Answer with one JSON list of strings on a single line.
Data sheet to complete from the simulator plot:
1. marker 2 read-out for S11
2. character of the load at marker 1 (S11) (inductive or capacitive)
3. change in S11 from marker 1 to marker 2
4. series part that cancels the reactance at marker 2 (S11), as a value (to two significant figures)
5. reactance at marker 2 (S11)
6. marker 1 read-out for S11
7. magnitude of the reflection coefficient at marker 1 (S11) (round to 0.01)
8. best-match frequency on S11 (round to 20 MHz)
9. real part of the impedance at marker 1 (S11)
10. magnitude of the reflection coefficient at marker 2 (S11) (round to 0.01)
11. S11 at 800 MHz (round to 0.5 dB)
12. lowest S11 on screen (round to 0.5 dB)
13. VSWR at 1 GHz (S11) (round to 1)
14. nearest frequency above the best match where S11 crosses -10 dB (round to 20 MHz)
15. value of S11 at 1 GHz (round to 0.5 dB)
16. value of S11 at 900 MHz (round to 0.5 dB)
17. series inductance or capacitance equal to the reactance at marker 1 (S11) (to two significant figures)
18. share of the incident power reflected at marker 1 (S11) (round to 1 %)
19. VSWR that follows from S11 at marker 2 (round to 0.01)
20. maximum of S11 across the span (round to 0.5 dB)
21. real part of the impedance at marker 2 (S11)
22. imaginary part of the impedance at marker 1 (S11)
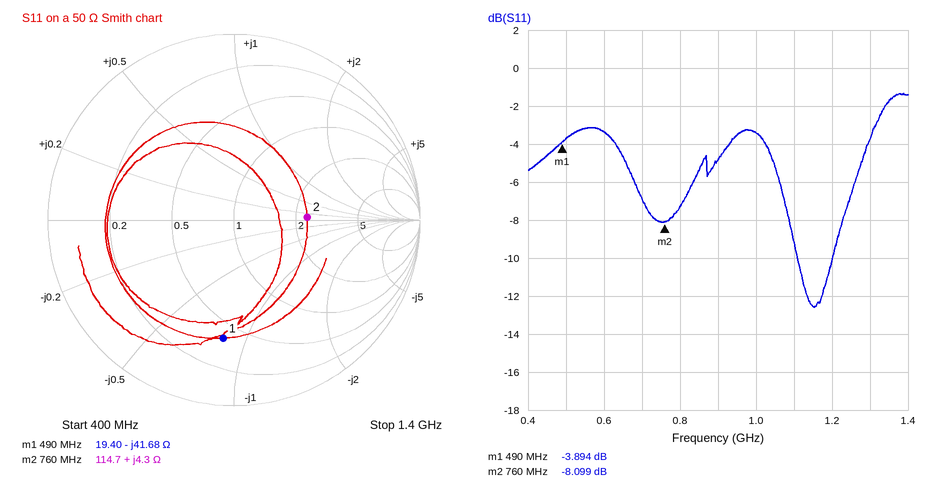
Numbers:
["-8.099 dB", "capacitive", "-4.205 dB", "49 pF", "+4.3 Ω", "-3.894 dB", "0.64", "1.16 GHz", "19.40 Ω", "0.39", "-7.5 dB", "-12.5 dB", "5", "1.20 GHz", "-3.5 dB", "-5.0 dB", "7.8 pF", "41 %", "2.30", "-1.5 dB", "114.7 Ω", "-41.68 Ω"]
